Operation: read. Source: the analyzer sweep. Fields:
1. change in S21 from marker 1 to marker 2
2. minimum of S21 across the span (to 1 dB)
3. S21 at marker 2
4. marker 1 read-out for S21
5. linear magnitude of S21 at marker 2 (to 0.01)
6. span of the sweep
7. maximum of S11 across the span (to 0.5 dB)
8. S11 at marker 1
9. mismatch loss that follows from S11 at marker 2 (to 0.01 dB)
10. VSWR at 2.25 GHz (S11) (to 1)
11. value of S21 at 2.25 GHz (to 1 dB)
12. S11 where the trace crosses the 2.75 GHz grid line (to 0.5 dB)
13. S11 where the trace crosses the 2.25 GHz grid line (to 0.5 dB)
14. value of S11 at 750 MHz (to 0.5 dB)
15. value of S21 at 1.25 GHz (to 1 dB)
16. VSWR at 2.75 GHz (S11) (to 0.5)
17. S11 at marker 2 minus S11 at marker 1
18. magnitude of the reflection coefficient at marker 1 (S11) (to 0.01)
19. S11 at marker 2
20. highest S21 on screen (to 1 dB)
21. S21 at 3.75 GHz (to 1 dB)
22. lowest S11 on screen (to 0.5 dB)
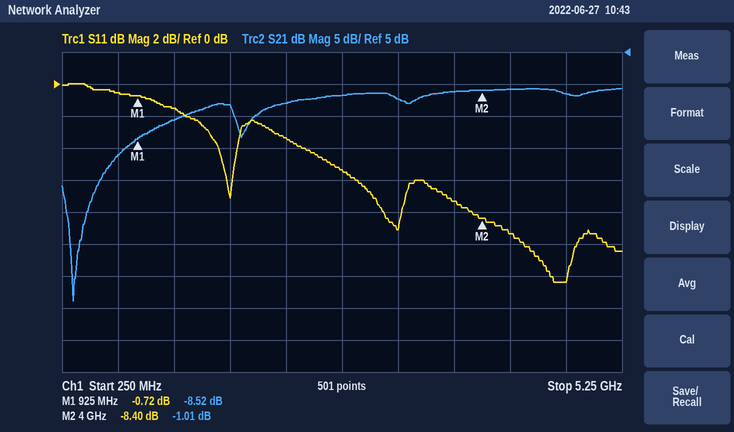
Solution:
7.51 dB
-34 dB
-1.01 dB
-8.52 dB
0.89
5 GHz
0.0 dB
-0.72 dB
0.68 dB
5
-3 dB
-5.5 dB
-3.5 dB
-0.5 dB
-6 dB
3.5
-7.68 dB
0.92
-8.40 dB
-1 dB
-1 dB
-12.5 dB
